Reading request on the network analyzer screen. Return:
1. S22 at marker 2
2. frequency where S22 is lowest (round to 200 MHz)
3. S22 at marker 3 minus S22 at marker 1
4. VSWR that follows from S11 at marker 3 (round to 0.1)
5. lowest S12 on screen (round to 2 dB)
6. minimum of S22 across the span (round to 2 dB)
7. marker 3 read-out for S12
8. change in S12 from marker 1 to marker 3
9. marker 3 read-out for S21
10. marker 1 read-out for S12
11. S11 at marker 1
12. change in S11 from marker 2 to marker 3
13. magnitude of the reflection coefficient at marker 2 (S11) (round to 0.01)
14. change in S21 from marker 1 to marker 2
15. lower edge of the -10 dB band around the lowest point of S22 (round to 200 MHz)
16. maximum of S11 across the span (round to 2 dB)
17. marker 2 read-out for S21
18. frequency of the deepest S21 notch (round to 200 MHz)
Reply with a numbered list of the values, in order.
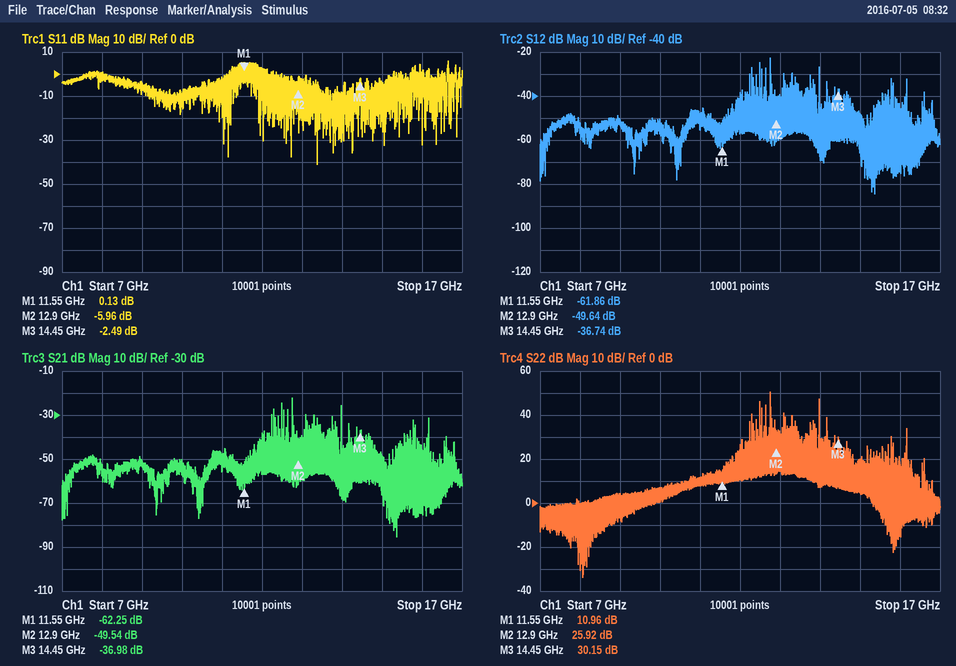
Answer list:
1. 25.92 dB
2. 8.0 GHz
3. 19.19 dB
4. 7.0
5. -84 dB
6. -34 dB
7. -36.74 dB
8. 25.12 dB
9. -36.98 dB
10. -61.86 dB
11. 0.13 dB
12. 3.47 dB
13. 0.50
14. 12.71 dB
15. 8.0 GHz
16. 6 dB
17. -49.54 dB
18. 15.4 GHz
